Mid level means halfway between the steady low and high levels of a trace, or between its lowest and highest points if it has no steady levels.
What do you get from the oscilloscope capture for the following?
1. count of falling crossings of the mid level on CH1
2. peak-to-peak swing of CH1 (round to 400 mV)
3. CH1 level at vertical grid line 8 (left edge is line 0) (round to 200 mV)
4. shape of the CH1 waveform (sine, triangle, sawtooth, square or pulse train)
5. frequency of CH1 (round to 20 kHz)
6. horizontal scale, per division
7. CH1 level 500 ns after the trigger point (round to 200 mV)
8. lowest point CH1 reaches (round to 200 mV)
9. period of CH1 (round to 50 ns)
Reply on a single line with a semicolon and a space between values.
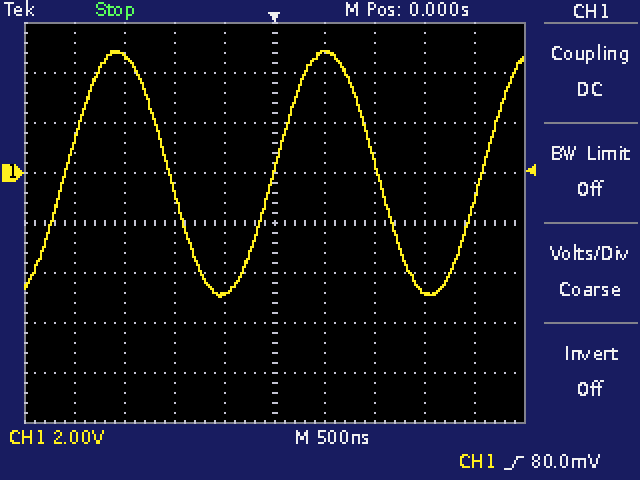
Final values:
2; 10.0 V; -4.8 V; sine; 480 kHz; 500 ns; 4.8 V; -5.0 V; 2.10 µs
